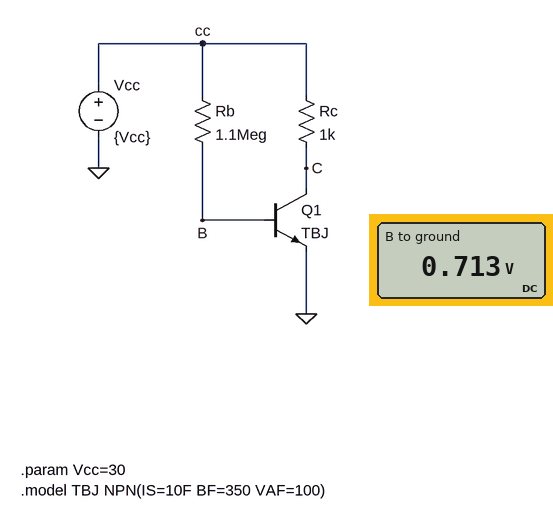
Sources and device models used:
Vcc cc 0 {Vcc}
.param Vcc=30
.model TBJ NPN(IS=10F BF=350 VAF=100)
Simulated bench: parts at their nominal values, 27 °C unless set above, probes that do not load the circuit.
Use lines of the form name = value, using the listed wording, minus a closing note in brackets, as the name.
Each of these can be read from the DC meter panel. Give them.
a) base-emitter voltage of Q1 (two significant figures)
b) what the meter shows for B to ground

base-emitter voltage of Q1 = 710 mV
what the meter shows for B to ground = 0.713 V
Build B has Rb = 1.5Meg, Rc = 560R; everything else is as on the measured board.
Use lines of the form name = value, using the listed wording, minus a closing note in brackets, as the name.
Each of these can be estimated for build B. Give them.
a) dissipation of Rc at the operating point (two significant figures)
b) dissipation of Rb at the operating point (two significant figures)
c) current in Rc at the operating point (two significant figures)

dissipation of Rc at the operating point = 41 mW
dissipation of Rb at the operating point = 570 µW
current in Rc at the operating point = 8.5 mA
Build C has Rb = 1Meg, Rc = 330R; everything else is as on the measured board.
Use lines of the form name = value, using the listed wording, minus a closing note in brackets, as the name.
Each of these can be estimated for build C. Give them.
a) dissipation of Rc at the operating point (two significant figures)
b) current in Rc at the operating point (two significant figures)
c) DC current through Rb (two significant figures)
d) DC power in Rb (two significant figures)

dissipation of Rc at the operating point = 54 mW
current in Rc at the operating point = 13 mA
DC current through Rb = 29 µA
DC power in Rb = 860 µW
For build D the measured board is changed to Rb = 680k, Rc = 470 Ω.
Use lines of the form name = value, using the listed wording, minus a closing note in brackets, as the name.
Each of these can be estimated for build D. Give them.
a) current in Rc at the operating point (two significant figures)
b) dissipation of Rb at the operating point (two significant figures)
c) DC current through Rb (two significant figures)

current in Rc at the operating point = 18 mA
dissipation of Rb at the operating point = 1.3 mW
DC current through Rb = 43 µA
